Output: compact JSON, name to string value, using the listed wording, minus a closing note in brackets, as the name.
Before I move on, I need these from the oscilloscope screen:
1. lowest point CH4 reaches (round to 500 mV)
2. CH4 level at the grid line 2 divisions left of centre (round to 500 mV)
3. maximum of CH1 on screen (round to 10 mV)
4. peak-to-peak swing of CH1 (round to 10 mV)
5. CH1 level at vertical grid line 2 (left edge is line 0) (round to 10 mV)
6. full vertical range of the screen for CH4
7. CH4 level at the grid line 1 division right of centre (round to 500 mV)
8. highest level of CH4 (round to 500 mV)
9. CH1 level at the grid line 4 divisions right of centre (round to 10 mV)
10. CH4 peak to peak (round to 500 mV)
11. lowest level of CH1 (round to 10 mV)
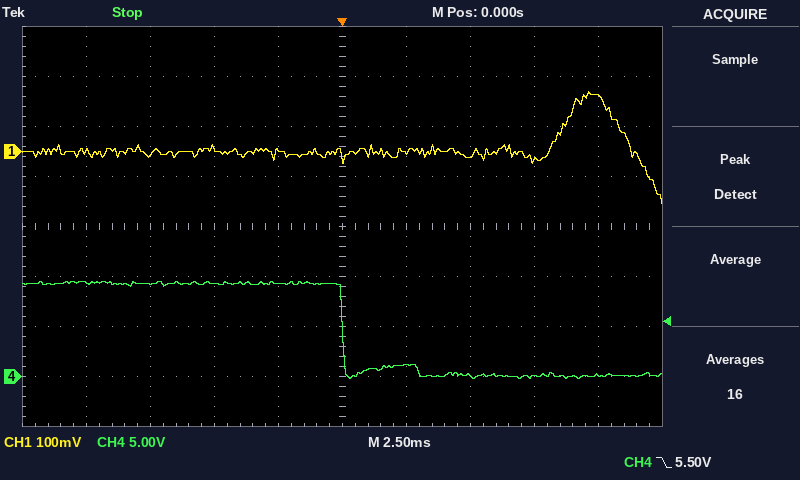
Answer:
{"lowest point CH4 reaches": "0.0 V", "CH4 level at the grid line 2 divisions left of centre": "9.5 V", "maximum of CH1 on screen": "120 mV", "peak-to-peak swing of CH1": "220 mV", "CH1 level at vertical grid line 2 (left edge is line 0)": "-10 mV", "full vertical range of the screen for CH4": "40 V", "CH4 level at the grid line 1 division right of centre": "1.0 V", "highest level of CH4": "9.5 V", "CH1 level at the grid line 4 divisions right of centre": "110 mV", "CH4 peak to peak": "9.5 V", "lowest level of CH1": "-100 mV"}
